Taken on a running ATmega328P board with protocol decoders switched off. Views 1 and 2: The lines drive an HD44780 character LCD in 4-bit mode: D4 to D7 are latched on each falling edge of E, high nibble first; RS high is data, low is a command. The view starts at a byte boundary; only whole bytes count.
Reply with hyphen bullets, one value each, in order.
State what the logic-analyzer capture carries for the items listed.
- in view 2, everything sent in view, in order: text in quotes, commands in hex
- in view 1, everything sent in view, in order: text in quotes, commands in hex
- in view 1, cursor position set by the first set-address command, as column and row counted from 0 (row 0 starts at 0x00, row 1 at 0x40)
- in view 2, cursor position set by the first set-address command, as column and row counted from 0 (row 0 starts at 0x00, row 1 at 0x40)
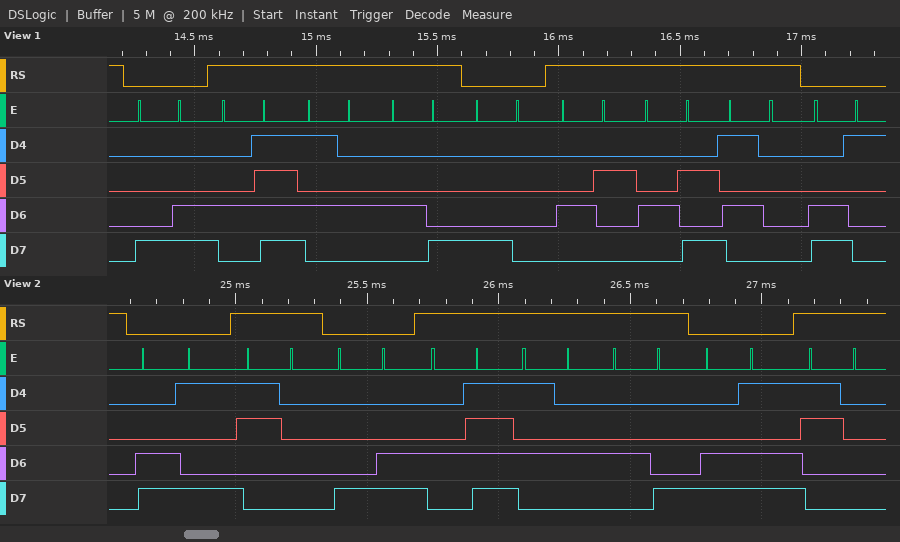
- 0xC9 "0" 0x8C "OTH" 0xCD "0"
- 0x8C "OTH" 0x80 "BJP" 0xC1
- column 12, row 0
- column 9, row 1
